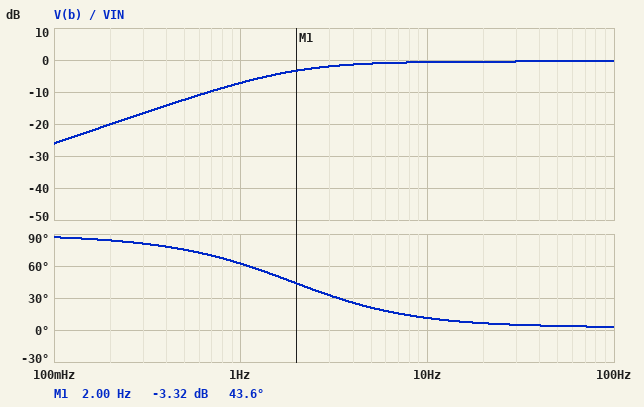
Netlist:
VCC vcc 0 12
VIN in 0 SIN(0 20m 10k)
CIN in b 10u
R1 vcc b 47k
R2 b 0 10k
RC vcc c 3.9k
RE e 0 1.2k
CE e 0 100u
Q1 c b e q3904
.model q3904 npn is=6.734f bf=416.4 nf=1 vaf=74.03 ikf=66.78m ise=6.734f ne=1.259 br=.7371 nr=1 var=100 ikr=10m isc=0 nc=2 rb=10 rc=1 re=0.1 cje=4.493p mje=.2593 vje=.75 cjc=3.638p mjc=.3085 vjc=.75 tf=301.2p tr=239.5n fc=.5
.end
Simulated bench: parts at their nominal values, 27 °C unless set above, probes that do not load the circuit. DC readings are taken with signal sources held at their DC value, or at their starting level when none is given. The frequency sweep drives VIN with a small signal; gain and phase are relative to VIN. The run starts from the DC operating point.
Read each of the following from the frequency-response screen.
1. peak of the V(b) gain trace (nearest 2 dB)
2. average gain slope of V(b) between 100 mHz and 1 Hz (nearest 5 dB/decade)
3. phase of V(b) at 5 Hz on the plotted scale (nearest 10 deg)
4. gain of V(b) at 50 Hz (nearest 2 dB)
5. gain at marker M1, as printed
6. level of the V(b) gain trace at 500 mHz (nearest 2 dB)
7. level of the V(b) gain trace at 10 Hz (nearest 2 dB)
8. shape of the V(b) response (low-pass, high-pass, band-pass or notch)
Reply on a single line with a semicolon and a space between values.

0 dB; 20 dB/decade; 20 deg; 0 dB; -3.32 dB; -12 dB; 0 dB; high-pass
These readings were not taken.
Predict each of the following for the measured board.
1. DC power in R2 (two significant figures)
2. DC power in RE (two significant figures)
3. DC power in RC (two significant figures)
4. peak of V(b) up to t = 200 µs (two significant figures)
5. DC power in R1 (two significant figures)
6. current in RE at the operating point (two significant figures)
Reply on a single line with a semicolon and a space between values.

420 µW; 1.6 mW; 5.0 mW; 2.1 V; 2.1 mW; 1.1 mA
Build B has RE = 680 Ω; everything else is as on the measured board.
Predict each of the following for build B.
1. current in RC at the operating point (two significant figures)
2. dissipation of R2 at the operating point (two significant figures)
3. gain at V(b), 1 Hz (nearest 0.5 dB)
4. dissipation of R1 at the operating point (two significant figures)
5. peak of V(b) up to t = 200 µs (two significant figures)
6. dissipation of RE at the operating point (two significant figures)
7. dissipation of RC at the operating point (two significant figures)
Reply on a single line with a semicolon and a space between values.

1.9 mA; 400 µW; -7.5 dB; 2.1 mW; 2.0 V; 2.5 mW; 14 mW
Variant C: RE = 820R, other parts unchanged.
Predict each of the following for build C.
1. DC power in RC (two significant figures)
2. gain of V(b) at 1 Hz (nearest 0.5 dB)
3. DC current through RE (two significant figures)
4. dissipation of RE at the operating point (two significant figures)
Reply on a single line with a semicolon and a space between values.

10 mW; -7.5 dB; 1.6 mA; 2.2 mW
